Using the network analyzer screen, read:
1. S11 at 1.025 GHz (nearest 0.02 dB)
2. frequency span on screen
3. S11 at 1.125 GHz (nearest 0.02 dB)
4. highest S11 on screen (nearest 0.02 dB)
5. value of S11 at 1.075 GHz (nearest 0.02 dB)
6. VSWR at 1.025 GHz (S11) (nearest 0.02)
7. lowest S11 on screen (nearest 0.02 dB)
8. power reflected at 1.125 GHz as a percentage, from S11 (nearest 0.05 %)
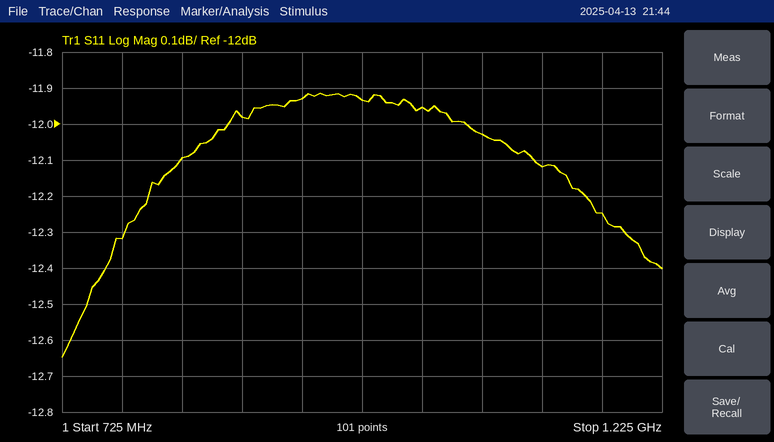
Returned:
-11.96 dB
500 MHz
-12.12 dB
-11.92 dB
-12.02 dB
1.68
-12.64 dB
6.15 %
